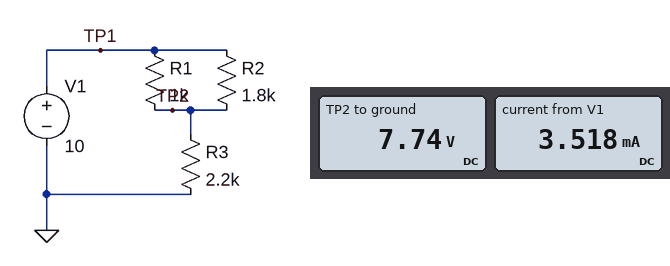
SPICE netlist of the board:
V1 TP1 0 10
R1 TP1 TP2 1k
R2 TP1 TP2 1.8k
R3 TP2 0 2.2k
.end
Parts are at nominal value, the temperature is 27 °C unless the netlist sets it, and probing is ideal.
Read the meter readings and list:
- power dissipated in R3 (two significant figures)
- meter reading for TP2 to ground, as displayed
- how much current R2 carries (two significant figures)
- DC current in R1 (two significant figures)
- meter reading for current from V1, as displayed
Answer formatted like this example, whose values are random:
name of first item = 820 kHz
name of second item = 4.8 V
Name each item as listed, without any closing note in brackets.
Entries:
power dissipated in R3 = 27 mW
meter reading for TP2 to ground, as displayed = 7.74 V
how much current R2 carries = 1.3 mA
DC current in R1 = 2.3 mA
meter reading for current from V1, as displayed = 3.518 mA
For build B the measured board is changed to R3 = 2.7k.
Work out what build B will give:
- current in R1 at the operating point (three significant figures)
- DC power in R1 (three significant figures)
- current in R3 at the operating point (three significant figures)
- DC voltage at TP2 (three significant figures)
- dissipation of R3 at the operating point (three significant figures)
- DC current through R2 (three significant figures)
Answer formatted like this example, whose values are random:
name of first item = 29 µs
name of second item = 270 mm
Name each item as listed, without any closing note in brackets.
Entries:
current in R1 at the operating point = 1.92 mA
DC power in R1 = 3.70 mW
current in R3 at the operating point = 2.99 mA
DC voltage at TP2 = 8.08 V
dissipation of R3 at the operating point = 24.2 mW
DC current through R2 = 1.07 mA
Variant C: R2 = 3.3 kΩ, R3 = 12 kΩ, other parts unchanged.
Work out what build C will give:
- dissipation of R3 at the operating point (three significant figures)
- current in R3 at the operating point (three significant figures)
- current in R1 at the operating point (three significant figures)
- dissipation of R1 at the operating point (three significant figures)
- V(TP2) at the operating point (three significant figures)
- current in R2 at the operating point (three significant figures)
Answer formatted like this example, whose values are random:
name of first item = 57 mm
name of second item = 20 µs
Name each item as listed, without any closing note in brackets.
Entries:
dissipation of R3 at the operating point = 7.36 mW
current in R3 at the operating point = 783 µA
current in R1 at the operating point = 601 µA
dissipation of R1 at the operating point = 361 µW
V(TP2) at the operating point = 9.40 V
current in R2 at the operating point = 182 µA
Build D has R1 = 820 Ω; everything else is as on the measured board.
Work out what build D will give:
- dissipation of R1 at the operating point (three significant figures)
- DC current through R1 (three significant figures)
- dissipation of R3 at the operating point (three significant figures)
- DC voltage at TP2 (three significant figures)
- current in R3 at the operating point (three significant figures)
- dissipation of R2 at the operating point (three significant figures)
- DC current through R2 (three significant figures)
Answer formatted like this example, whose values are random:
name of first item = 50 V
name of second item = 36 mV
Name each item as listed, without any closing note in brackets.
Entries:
dissipation of R1 at the operating point = 5.07 mW
DC current through R1 = 2.49 mA
dissipation of R3 at the operating point = 28.8 mW
DC voltage at TP2 = 7.96 V
current in R3 at the operating point = 3.62 mA
dissipation of R2 at the operating point = 2.31 mW
DC current through R2 = 1.13 mA
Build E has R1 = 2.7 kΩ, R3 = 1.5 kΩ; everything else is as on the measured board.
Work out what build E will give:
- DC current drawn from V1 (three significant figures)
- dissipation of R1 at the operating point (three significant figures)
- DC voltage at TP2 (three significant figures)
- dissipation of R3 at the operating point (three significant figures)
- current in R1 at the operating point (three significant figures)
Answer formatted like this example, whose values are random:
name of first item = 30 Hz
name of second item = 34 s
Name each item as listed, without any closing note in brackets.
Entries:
DC current drawn from V1 = 3.88 mA
dissipation of R1 at the operating point = 6.49 mW
DC voltage at TP2 = 5.81 V
dissipation of R3 at the operating point = 22.5 mW
current in R1 at the operating point = 1.55 mA
